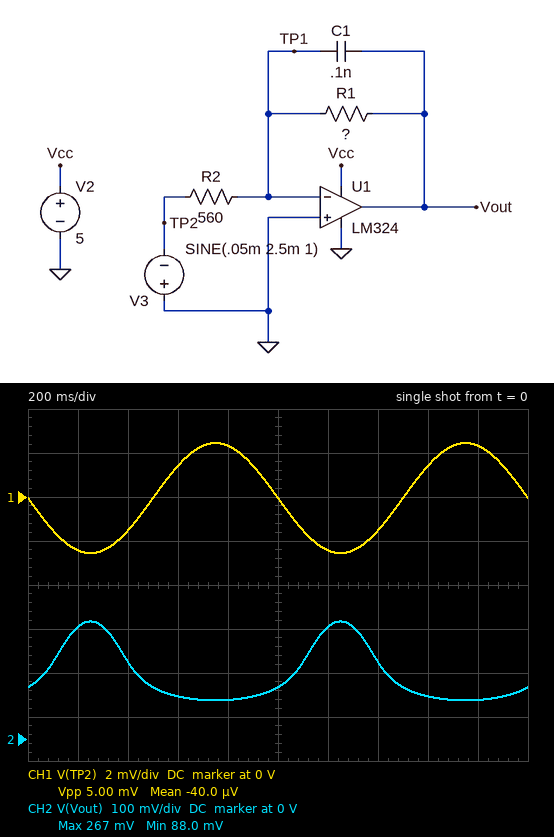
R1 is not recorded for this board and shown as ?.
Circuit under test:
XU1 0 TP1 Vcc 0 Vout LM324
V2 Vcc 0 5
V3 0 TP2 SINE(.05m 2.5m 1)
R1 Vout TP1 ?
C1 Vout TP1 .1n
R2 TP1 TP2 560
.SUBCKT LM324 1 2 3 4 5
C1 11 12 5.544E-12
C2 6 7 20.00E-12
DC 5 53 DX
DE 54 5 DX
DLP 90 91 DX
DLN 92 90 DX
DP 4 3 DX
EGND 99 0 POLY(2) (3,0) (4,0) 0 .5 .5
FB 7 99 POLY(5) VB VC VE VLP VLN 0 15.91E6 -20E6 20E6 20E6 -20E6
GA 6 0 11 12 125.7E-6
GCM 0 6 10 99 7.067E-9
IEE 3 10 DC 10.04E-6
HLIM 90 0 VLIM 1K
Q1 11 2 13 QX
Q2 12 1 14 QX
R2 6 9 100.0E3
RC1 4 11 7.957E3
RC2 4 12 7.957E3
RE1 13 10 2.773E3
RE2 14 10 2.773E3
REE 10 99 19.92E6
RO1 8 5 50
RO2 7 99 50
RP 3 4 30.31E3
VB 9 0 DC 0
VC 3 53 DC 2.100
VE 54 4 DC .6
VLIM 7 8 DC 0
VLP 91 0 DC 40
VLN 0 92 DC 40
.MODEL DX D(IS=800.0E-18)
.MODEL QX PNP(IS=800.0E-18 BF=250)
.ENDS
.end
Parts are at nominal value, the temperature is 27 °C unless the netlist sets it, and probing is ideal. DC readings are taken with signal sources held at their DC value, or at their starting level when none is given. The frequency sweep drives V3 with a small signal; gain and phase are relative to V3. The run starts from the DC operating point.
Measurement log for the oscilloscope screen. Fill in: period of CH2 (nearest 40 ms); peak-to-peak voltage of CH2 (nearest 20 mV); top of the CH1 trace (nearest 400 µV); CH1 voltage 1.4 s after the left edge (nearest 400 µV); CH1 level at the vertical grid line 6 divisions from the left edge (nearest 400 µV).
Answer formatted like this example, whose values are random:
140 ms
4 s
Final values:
1.00 s
180 mV
2.4 mV
-1.6 mV
-2.4 mV
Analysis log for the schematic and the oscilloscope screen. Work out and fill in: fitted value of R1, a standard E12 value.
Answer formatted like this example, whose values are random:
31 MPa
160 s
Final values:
56 kΩ
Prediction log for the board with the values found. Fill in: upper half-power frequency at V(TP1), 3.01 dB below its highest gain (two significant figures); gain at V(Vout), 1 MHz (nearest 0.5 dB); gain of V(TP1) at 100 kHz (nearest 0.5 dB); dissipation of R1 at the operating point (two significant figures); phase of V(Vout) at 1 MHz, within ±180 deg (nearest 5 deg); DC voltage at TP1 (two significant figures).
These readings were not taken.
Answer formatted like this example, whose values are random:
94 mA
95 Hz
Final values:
3.9 MHz
-6.0 dB
-2.0 dB
240 nW
-130 deg
1.1 mV
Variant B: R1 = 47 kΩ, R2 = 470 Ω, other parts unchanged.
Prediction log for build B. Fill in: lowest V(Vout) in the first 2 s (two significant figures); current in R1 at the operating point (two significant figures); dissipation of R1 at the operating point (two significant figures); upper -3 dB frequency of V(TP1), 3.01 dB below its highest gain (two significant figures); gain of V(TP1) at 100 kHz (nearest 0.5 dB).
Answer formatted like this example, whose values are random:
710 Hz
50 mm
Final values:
88 mV
2.5 µA
290 nW
4.4 MHz
-1.5 dB
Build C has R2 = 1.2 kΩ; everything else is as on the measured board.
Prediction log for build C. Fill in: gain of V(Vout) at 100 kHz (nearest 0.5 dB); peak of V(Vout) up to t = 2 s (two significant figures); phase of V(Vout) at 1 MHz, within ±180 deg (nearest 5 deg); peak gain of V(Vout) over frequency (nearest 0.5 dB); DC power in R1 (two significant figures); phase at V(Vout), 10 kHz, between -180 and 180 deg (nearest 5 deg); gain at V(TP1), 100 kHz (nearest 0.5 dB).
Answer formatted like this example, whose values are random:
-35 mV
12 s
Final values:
10.5 dB
140 mV
-140 deg
20.0 dB
170 nW
-15 deg
-3.0 dB
